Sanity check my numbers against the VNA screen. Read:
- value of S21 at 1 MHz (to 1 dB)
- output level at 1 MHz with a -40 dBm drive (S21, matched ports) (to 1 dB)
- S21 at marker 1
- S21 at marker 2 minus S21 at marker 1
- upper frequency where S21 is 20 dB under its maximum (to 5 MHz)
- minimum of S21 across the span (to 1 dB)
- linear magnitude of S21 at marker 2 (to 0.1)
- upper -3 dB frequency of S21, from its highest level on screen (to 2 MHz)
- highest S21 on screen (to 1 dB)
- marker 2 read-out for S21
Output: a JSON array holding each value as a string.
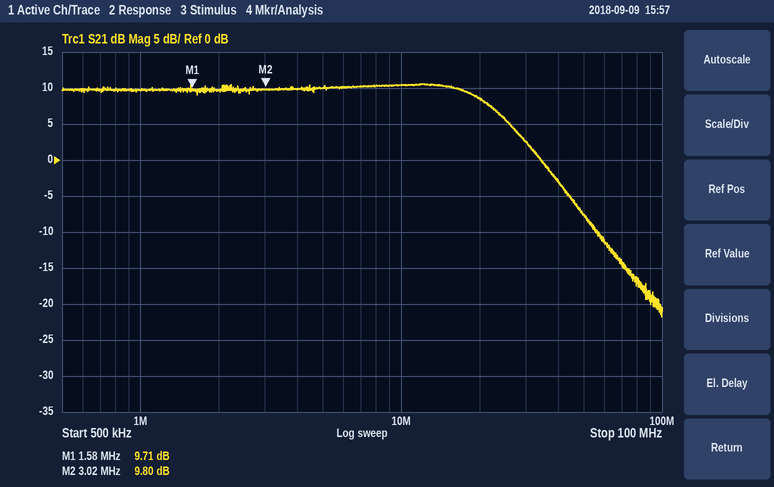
["10 dB", "-30 dBm", "9.71 dB", "0.09 dB", "55 MHz", "-22 dB", "3.1", "22 MHz", "11 dB", "9.80 dB"]
